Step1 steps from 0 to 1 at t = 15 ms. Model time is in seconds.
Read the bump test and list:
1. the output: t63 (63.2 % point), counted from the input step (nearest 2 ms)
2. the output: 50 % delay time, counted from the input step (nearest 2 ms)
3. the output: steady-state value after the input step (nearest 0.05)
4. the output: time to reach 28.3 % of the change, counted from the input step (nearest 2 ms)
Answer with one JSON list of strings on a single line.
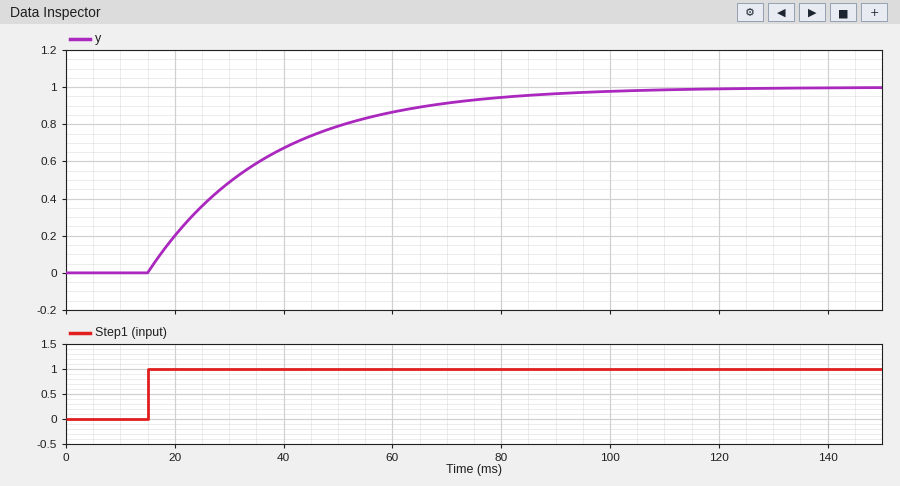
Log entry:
["22 ms", "16 ms", "1.00", "8 ms"]
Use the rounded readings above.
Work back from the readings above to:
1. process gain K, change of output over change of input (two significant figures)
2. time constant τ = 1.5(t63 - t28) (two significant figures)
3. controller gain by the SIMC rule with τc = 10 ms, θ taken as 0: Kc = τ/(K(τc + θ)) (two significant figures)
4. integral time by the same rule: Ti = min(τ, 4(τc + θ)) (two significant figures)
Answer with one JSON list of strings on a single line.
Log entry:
["1.0", "21 ms", "2.1", "21 ms"]
